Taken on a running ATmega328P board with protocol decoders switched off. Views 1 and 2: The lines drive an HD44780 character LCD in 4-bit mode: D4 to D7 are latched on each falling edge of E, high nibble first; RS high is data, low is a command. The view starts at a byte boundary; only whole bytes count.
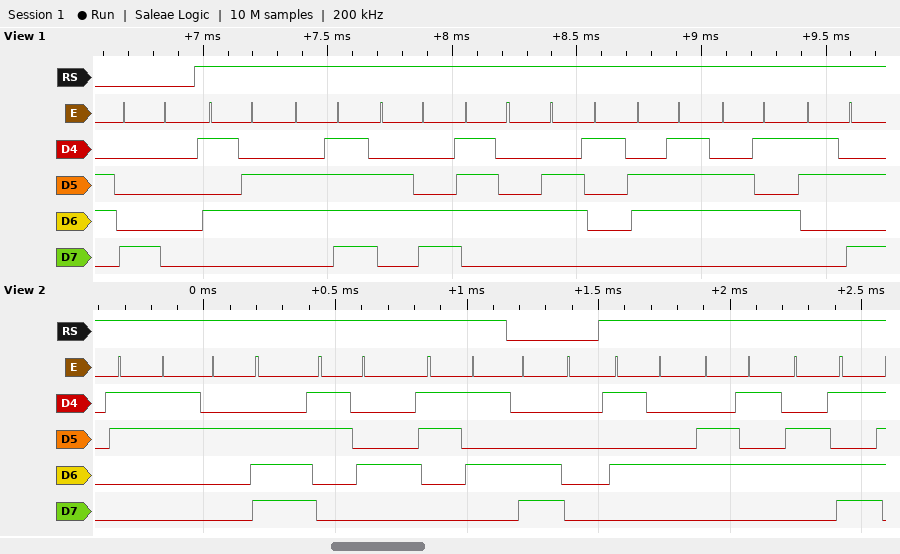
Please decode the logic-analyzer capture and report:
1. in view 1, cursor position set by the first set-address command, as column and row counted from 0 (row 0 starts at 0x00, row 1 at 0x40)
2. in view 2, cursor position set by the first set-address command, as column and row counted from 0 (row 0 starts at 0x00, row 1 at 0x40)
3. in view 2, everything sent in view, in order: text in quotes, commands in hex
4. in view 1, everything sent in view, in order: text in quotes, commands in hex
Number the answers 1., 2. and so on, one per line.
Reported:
1. column 0, row 0
2. column 0, row 1
3. "3.45" 0xC0 "Tem"
4. 0x80 "Voltage:"
